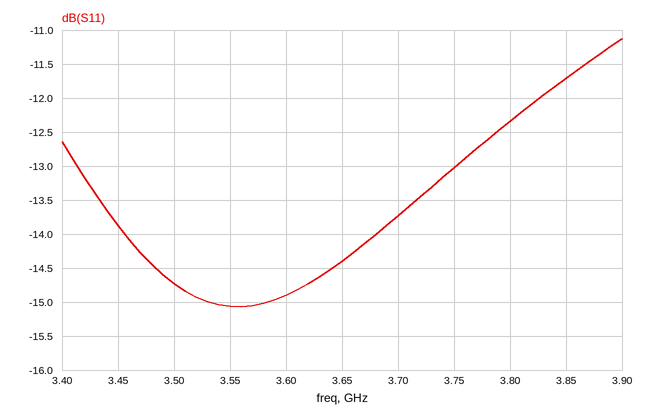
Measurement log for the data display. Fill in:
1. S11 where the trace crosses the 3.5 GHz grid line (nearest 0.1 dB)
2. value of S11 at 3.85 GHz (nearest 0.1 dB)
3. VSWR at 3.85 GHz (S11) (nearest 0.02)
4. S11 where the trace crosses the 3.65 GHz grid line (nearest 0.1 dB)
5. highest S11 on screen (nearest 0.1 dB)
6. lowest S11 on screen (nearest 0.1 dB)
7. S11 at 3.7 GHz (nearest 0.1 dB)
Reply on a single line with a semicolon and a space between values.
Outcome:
-14.7 dB; -11.7 dB; 1.70; -14.4 dB; -11.1 dB; -15.1 dB; -13.7 dB
